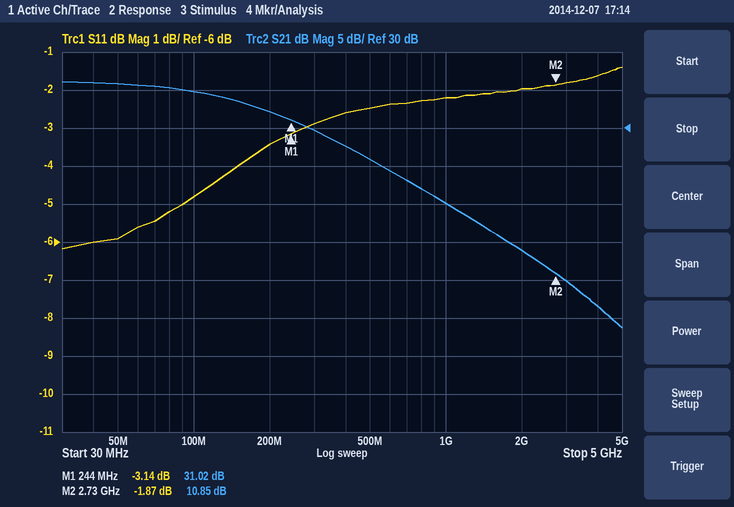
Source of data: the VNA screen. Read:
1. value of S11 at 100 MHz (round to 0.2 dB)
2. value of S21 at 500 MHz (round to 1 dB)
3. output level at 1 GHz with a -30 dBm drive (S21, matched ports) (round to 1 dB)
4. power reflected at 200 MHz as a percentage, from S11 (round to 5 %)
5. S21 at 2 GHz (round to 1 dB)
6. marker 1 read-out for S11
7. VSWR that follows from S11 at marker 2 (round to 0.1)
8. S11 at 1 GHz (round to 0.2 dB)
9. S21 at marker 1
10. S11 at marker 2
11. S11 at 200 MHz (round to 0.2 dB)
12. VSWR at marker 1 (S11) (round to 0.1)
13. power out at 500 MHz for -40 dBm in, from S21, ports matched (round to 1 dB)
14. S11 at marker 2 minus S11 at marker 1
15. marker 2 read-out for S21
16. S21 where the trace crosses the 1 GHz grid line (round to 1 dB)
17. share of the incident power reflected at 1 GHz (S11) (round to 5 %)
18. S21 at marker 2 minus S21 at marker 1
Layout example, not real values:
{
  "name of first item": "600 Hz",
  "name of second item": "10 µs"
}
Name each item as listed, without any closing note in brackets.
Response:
{
  "value of S11 at 100 MHz": "-4.8 dB",
  "value of S21 at 500 MHz": "26 dB",
  "output level at 1 GHz with a -30 dBm drive (S21, matched ports)": "-10 dBm",
  "power reflected at 200 MHz as a percentage, from S11": "45 %",
  "S21 at 2 GHz": "14 dB",
  "marker 1 read-out for S11": "-3.14 dB",
  "VSWR that follows from S11 at marker 2": "9.3",
  "S11 at 1 GHz": "-2.2 dB",
  "S21 at marker 1": "31.02 dB",
  "S11 at marker 2": "-1.87 dB",
  "S11 at 200 MHz": "-3.4 dB",
  "VSWR at marker 1 (S11)": "5.6",
  "power out at 500 MHz for -40 dBm in, from S21, ports matched": "-14 dBm",
  "S11 at marker 2 minus S11 at marker 1": "1.27 dB",
  "marker 2 read-out for S21": "10.85 dB",
  "S21 where the trace crosses the 1 GHz grid line": "20 dB",
  "share of the incident power reflected at 1 GHz (S11)": "60 %",
  "S21 at marker 2 minus S21 at marker 1": "-20.17 dB"
}
